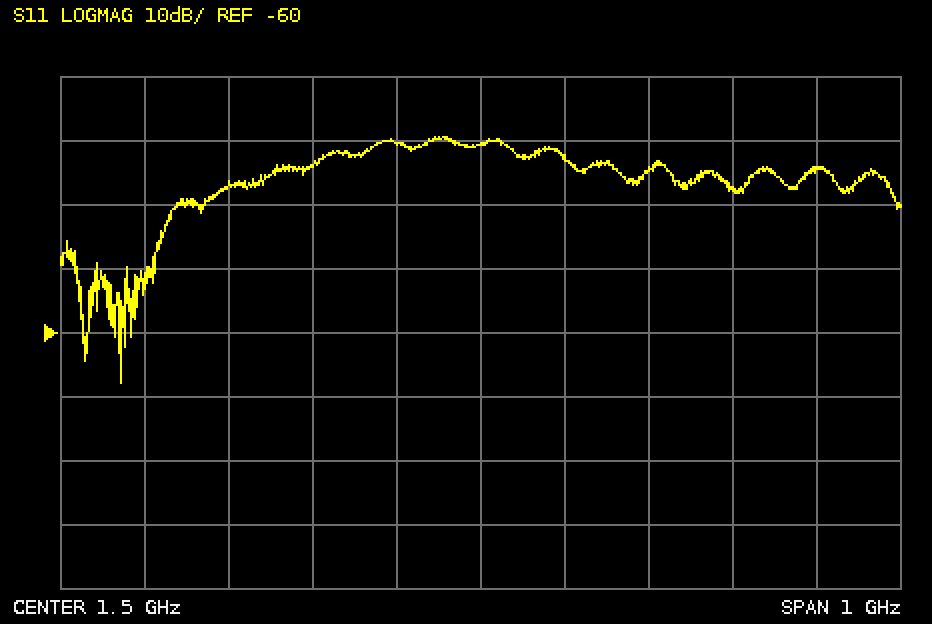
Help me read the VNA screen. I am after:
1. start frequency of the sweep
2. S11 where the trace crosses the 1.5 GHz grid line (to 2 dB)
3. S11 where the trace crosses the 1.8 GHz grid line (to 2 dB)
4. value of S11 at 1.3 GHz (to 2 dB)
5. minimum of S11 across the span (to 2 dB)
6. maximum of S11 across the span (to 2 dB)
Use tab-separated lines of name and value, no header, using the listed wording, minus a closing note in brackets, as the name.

start frequency of the sweep	1 GHz
S11 where the trace crosses the 1.5 GHz grid line	-30 dB
S11 where the trace crosses the 1.8 GHz grid line	-38 dB
value of S11 at 1.3 GHz	-34 dB
minimum of S11 across the span	-68 dB
maximum of S11 across the span	-30 dB
